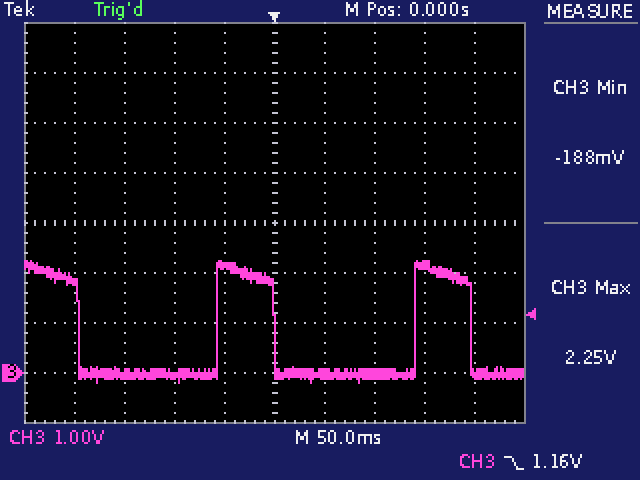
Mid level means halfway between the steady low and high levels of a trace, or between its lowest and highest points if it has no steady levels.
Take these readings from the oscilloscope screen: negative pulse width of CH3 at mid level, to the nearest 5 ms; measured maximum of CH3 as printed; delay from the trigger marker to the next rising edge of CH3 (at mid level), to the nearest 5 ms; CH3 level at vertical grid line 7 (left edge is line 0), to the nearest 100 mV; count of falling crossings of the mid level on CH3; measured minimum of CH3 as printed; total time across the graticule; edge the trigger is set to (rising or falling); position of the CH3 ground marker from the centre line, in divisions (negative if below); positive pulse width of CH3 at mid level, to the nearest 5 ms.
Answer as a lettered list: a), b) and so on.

a) 140 ms
b) 2.25 V
c) 140 ms
d) 0.0 V
e) 3
f) -188 mV
g) 500 ms
h) falling
i) -3.0 div
j) 55 ms
